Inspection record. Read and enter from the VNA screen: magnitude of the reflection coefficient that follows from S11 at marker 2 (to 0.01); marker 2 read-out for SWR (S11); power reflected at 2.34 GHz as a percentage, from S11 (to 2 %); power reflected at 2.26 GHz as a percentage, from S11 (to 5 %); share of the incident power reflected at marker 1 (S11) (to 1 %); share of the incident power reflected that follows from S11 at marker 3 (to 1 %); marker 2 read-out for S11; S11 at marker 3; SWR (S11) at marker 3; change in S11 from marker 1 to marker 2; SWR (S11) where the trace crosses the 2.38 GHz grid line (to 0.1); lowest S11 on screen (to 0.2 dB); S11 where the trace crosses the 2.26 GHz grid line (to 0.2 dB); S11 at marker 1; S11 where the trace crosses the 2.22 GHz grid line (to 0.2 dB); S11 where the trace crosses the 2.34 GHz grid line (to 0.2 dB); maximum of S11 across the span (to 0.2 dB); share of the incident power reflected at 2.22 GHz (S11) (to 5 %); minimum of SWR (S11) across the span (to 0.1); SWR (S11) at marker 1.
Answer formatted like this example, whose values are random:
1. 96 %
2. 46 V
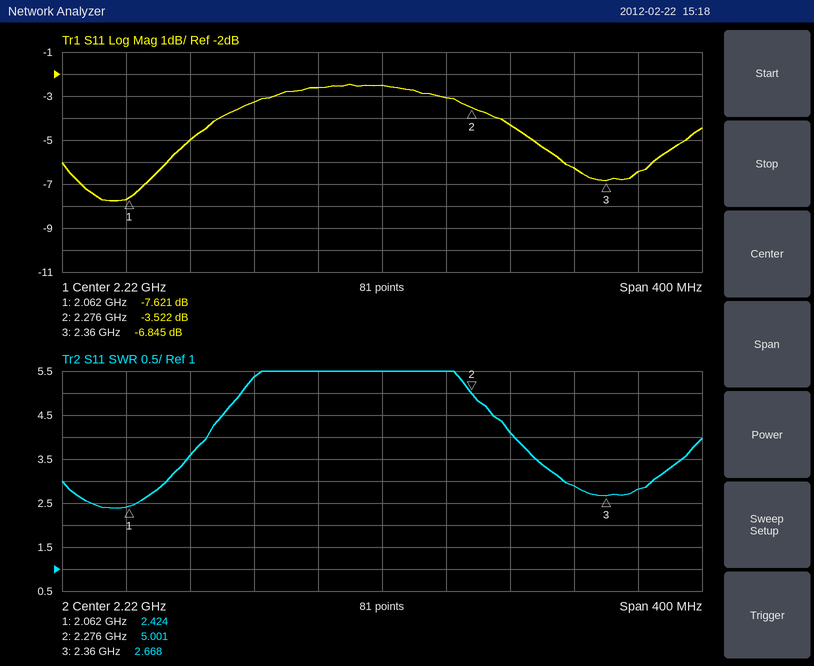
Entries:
1. 0.67
2. 5.001
3. 24 %
4. 50 %
5. 17 %
6. 21 %
7. -3.522 dB
8. -6.845 dB
9. 2.668
10. 4.099 dB
11. 2.8
12. -7.8 dB
13. -3.0 dB
14. -7.621 dB
15. -2.6 dB
16. -6.2 dB
17. -2.4 dB
18. 55 %
19. 2.4
20. 2.424
